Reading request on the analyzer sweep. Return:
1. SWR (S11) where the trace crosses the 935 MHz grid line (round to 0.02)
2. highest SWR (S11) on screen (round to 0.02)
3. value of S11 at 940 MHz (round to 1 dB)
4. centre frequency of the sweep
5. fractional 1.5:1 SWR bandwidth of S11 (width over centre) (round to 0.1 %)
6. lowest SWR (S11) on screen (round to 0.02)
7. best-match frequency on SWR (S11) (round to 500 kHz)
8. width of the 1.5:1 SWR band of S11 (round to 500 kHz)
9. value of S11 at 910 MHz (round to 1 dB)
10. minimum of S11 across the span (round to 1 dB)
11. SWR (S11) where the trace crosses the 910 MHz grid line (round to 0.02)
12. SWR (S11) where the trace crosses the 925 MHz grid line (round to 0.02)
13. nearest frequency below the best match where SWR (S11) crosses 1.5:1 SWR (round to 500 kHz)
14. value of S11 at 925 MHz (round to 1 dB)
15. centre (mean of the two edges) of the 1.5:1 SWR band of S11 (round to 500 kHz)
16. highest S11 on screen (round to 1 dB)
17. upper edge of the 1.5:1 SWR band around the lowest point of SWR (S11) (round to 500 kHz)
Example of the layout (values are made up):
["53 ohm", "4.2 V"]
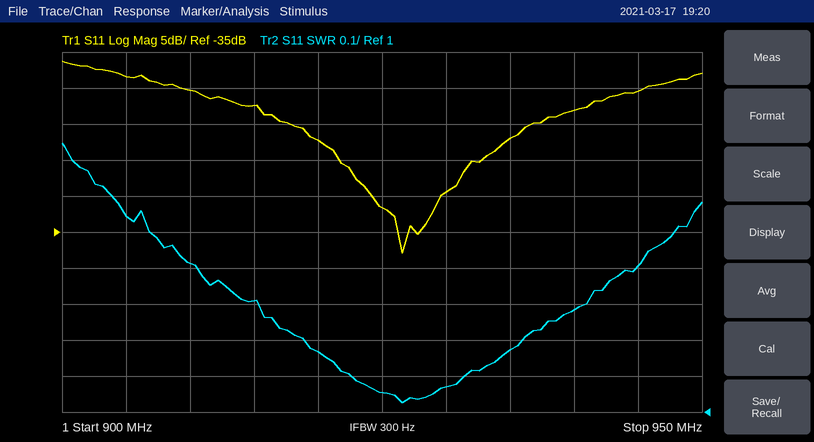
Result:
["1.18", "1.74", "-18 dB", "925 MHz", "4.4 %", "1.02", "926.5 MHz", "41.0 MHz", "-15 dB", "-38 dB", "1.42", "1.06", "907.0 MHz", "-32 dB", "927.5 MHz", "-11 dB", "948.0 MHz"]
